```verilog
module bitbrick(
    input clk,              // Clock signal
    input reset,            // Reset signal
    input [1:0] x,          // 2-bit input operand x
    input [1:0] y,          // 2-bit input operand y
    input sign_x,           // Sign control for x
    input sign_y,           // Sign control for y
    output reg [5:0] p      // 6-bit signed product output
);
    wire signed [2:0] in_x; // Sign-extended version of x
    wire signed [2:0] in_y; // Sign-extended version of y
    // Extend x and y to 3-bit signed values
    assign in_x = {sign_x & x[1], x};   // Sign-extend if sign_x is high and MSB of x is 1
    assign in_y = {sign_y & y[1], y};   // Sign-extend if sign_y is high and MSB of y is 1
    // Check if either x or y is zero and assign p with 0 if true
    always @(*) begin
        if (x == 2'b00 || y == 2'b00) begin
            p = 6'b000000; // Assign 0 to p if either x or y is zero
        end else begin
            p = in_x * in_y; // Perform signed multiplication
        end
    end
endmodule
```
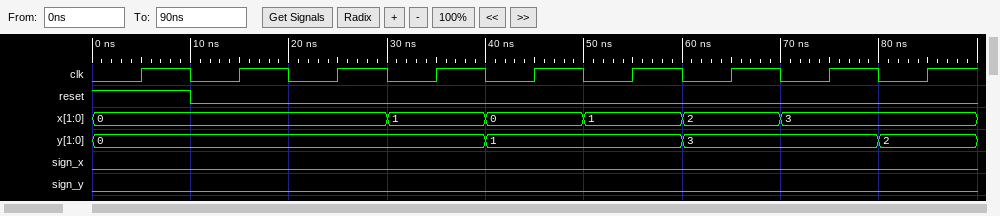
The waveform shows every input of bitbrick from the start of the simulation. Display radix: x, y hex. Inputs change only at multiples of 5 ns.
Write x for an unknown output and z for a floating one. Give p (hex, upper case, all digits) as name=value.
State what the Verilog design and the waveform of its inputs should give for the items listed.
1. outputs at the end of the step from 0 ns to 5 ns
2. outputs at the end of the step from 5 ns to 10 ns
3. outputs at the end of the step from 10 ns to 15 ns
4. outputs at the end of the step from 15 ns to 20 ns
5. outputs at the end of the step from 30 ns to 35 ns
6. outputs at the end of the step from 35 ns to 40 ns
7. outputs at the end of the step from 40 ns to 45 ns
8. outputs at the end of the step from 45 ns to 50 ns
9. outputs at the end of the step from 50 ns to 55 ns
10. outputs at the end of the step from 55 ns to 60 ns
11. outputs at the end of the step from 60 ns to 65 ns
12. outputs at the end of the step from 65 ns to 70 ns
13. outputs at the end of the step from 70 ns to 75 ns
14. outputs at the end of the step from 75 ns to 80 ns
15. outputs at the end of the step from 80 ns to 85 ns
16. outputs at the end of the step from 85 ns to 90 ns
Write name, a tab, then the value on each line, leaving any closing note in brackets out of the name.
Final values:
outputs at the end of the step from 0 ns to 5 ns	p=00
outputs at the end of the step from 5 ns to 10 ns	p=00
outputs at the end of the step from 10 ns to 15 ns	p=00
outputs at the end of the step from 15 ns to 20 ns	p=00
outputs at the end of the step from 30 ns to 35 ns	p=00
outputs at the end of the step from 35 ns to 40 ns	p=00
outputs at the end of the step from 40 ns to 45 ns	p=00
outputs at the end of the step from 45 ns to 50 ns	p=00
outputs at the end of the step from 50 ns to 55 ns	p=01
outputs at the end of the step from 55 ns to 60 ns	p=01
outputs at the end of the step from 60 ns to 65 ns	p=06
outputs at the end of the step from 65 ns to 70 ns	p=06
outputs at the end of the step from 70 ns to 75 ns	p=09
outputs at the end of the step from 75 ns to 80 ns	p=09
outputs at the end of the step from 80 ns to 85 ns	p=06
outputs at the end of the step from 85 ns to 90 ns	p=06
